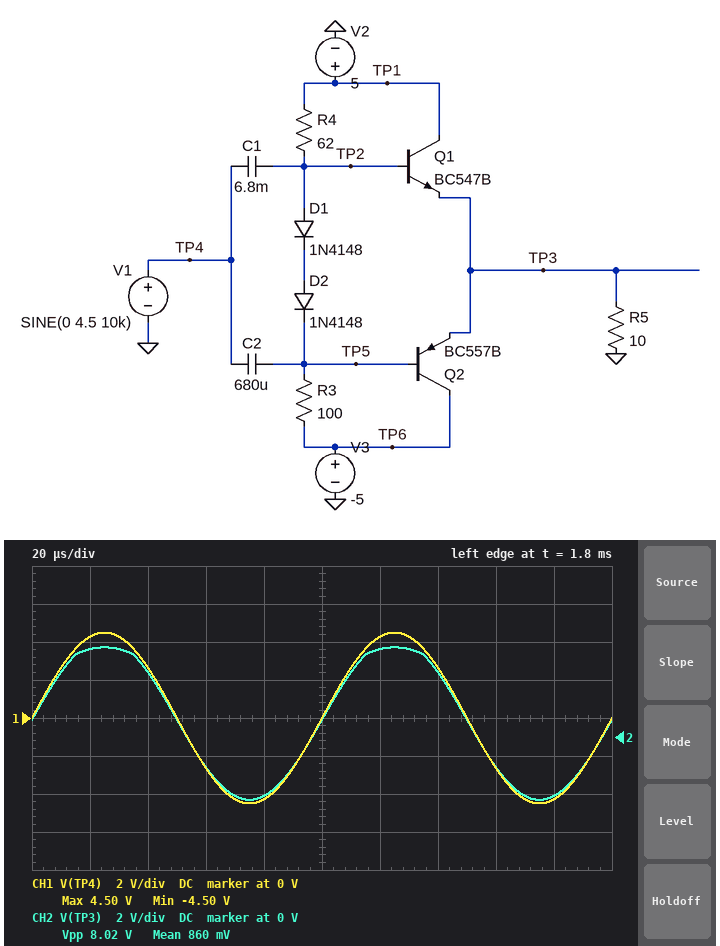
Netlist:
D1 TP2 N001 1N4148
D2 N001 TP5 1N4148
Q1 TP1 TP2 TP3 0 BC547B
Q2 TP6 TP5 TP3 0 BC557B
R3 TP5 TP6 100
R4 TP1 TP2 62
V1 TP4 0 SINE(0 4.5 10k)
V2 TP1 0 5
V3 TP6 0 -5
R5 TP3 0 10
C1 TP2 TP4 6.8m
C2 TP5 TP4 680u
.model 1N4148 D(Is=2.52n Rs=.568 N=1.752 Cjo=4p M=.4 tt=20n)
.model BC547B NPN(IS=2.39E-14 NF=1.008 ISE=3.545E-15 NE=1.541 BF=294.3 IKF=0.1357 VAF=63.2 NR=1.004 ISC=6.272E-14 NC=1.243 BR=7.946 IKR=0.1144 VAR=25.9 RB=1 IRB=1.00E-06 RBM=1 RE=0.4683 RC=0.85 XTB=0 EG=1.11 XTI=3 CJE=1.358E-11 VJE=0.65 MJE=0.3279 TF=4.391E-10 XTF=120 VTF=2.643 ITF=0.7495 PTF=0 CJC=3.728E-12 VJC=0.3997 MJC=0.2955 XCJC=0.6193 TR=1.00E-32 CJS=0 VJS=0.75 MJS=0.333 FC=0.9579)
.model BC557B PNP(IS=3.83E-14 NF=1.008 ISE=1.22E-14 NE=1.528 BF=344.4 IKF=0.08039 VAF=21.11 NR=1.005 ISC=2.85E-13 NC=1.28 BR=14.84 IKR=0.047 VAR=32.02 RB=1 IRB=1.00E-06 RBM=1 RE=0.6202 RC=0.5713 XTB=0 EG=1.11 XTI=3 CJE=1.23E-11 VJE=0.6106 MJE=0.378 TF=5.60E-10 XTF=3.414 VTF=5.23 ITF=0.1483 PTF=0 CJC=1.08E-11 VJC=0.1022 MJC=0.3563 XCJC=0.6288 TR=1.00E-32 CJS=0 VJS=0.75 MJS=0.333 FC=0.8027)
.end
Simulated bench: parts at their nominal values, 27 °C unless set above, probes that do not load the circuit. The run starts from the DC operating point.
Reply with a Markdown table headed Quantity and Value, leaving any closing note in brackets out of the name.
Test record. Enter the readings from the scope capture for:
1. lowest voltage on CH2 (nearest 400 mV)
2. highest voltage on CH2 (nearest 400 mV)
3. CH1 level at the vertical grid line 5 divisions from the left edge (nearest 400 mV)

| Quantity | Value |
|---|---|
| lowest voltage on CH2 | -3.2 V |
| highest voltage on CH2 | 4.8 V |
| CH1 level at the vertical grid line 5 divisions from the left edge | 0 V |
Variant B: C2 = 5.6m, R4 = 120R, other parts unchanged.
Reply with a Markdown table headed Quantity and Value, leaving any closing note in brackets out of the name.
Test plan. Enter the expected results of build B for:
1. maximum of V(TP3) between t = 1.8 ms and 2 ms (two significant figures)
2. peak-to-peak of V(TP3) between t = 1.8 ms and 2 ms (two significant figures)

| Quantity | Value |
|---|---|
| maximum of V(TP3) between t = 1.8 ms and 2 ms | 3.9 V |
| peak-to-peak of V(TP3) between t = 1.8 ms and 2 ms | 8.3 V |
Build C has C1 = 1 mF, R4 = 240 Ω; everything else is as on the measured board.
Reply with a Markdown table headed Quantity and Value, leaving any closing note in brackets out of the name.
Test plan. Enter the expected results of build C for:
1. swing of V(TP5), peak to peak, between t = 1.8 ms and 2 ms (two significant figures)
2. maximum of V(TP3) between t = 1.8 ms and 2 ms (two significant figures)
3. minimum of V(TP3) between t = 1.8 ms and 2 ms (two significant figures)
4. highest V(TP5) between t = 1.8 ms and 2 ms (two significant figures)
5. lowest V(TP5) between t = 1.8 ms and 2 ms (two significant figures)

| Quantity | Value |
|---|---|
| swing of V(TP5), peak to peak, between t = 1.8 ms and 2 ms | 9.0 V |
| maximum of V(TP3) between t = 1.8 ms and 2 ms | 2.7 V |
| minimum of V(TP3) between t = 1.8 ms and 2 ms | -4.8 V |
| highest V(TP5) between t = 1.8 ms and 2 ms | 2.4 V |
| lowest V(TP5) between t = 1.8 ms and 2 ms | -6.6 V |
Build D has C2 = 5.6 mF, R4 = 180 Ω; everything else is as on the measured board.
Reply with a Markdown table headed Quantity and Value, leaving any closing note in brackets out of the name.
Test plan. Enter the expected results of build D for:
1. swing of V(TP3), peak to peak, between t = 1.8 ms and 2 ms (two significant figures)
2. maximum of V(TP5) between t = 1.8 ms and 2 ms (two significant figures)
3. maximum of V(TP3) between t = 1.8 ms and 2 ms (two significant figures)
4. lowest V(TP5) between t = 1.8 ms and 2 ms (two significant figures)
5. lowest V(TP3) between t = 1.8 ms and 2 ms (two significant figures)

| Quantity | Value |
|---|---|
| swing of V(TP3), peak to peak, between t = 1.8 ms and 2 ms | 7.8 V |
| maximum of V(TP5) between t = 1.8 ms and 2 ms | 2.6 V |
| maximum of V(TP3) between t = 1.8 ms and 2 ms | 3.1 V |
| lowest V(TP5) between t = 1.8 ms and 2 ms | -6.4 V |
| lowest V(TP3) between t = 1.8 ms and 2 ms | -4.7 V |
